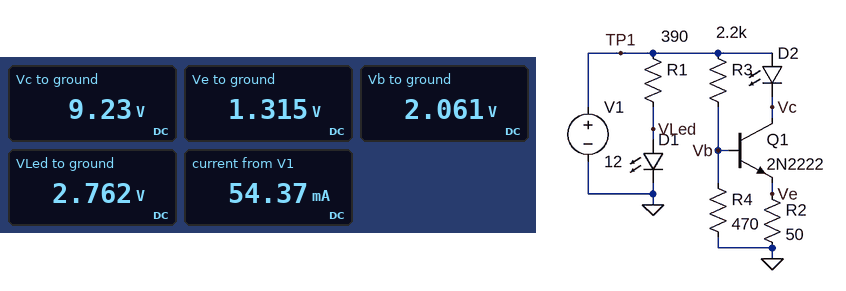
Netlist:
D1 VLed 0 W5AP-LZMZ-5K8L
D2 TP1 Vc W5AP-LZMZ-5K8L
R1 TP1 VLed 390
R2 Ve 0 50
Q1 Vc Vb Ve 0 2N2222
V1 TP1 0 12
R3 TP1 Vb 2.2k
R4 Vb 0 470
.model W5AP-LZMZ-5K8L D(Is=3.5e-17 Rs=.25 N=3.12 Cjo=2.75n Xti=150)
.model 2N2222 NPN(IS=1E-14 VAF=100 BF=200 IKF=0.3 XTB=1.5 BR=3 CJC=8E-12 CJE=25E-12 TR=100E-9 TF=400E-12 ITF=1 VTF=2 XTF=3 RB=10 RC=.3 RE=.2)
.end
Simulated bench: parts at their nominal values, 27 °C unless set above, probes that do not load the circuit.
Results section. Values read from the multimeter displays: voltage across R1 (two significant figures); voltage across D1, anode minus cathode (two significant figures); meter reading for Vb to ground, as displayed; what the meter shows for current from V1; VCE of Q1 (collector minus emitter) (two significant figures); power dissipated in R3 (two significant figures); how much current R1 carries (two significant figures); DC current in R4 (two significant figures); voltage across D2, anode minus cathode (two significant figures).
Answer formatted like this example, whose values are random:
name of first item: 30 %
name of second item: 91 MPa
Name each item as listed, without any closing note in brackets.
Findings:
voltage across R1: 9.2 V
voltage across D1, anode minus cathode: 2.8 V
meter reading for Vb to ground, as displayed: 2.061 V
what the meter shows for current from V1: 54.37 mA
VCE of Q1 (collector minus emitter): 7.9 V
power dissipated in R3: 45 mW
how much current R1 carries: 24 mA
DC current in R4: 4.4 mA
voltage across D2, anode minus cathode: 2.8 V
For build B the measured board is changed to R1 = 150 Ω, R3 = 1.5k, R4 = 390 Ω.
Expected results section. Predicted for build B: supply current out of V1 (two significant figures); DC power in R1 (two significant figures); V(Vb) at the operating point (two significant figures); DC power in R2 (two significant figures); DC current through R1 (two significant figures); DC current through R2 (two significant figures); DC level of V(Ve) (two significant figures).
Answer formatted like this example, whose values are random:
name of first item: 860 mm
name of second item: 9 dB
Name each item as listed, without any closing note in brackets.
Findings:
supply current out of V1: 100 mA
DC power in R1: 560 mW
V(Vb) at the operating point: 2.4 V
DC power in R2: 56 mW
DC current through R1: 61 mA
DC current through R2: 33 mA
DC level of V(Ve): 1.7 V
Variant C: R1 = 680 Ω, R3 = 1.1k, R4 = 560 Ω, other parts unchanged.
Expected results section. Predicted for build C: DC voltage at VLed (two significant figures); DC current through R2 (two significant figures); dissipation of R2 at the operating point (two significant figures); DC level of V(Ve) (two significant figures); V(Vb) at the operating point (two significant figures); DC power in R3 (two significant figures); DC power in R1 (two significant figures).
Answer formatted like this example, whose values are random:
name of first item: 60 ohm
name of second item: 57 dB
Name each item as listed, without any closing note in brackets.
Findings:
DC voltage at VLed: 2.7 V
DC current through R2: 63 mA
dissipation of R2 at the operating point: 200 mW
DC level of V(Ve): 3.1 V
V(Vb) at the operating point: 3.9 V
DC power in R3: 59 mW
DC power in R1: 130 mW
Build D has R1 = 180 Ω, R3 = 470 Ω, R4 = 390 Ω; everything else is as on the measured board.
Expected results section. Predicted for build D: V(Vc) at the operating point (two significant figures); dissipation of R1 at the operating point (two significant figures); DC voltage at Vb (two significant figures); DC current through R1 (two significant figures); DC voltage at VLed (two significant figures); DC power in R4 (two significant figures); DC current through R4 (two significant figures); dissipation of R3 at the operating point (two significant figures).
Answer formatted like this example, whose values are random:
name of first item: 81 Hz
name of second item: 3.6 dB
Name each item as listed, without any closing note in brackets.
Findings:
V(Vc) at the operating point: 9.1 V
dissipation of R1 at the operating point: 470 mW
DC voltage at Vb: 5.3 V
DC current through R1: 51 mA
DC voltage at VLed: 2.8 V
DC power in R4: 73 mW
DC current through R4: 14 mA
dissipation of R3 at the operating point: 95 mW
